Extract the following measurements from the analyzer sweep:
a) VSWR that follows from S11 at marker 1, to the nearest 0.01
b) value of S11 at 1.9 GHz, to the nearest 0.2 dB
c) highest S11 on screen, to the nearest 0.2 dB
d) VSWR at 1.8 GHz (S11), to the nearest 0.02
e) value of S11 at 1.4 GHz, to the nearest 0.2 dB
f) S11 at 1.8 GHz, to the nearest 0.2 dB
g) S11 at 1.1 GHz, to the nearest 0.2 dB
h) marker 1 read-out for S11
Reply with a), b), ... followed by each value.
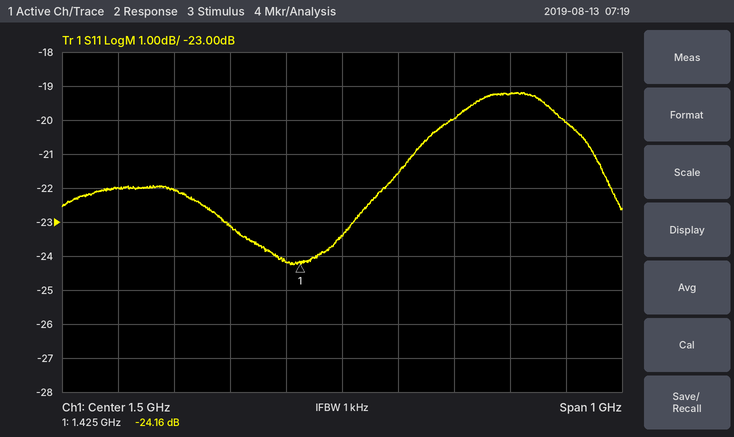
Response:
a) 1.13
b) -20.0 dB
c) -19.2 dB
d) 1.24
e) -24.2 dB
f) -19.2 dB
g) -22.0 dB
h) -24.16 dB
